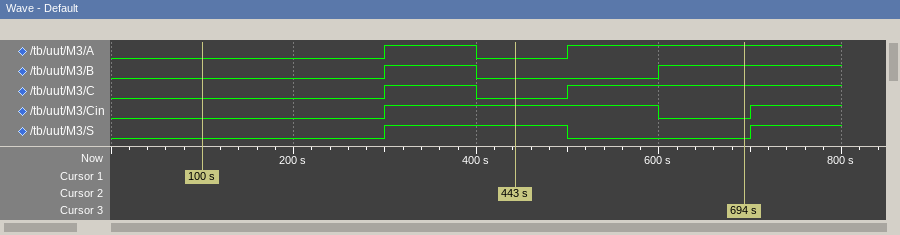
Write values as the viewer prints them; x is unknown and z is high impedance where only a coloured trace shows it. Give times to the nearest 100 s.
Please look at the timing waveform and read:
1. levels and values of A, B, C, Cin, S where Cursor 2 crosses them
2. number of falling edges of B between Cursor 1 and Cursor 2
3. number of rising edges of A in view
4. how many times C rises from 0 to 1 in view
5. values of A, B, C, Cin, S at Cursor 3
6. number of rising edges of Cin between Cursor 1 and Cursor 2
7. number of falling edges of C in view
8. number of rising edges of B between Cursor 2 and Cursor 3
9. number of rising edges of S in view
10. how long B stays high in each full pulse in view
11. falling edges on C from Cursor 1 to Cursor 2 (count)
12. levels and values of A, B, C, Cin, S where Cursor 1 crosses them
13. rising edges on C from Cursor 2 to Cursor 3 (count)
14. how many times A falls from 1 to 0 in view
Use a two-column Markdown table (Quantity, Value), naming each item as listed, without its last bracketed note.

| Quantity | Value |
|---|---|
| levels and values of A, B, C, Cin, S where Cursor 2 crosses them | A=0, B=0, C=0, Cin=1, S=1 |
| number of falling edges of B between Cursor 1 and Cursor 2 | 1 |
| number of rising edges of A in view | 2 |
| how many times C rises from 0 to 1 in view | 2 |
| values of A, B, C, Cin, S at Cursor 3 | A=1, B=1, C=1, Cin=0, S=0 |
| number of rising edges of Cin between Cursor 1 and Cursor 2 | 1 |
| number of falling edges of C in view | 1 |
| number of rising edges of B between Cursor 2 and Cursor 3 | 1 |
| number of rising edges of S in view | 2 |
| how long B stays high in each full pulse in view | 100 s |
| falling edges on C from Cursor 1 to Cursor 2 | 1 |
| levels and values of A, B, C, Cin, S where Cursor 1 crosses them | A=0, B=0, C=0, Cin=0, S=0 |
| rising edges on C from Cursor 2 to Cursor 3 | 1 |
| how many times A falls from 1 to 0 in view | 1 |
